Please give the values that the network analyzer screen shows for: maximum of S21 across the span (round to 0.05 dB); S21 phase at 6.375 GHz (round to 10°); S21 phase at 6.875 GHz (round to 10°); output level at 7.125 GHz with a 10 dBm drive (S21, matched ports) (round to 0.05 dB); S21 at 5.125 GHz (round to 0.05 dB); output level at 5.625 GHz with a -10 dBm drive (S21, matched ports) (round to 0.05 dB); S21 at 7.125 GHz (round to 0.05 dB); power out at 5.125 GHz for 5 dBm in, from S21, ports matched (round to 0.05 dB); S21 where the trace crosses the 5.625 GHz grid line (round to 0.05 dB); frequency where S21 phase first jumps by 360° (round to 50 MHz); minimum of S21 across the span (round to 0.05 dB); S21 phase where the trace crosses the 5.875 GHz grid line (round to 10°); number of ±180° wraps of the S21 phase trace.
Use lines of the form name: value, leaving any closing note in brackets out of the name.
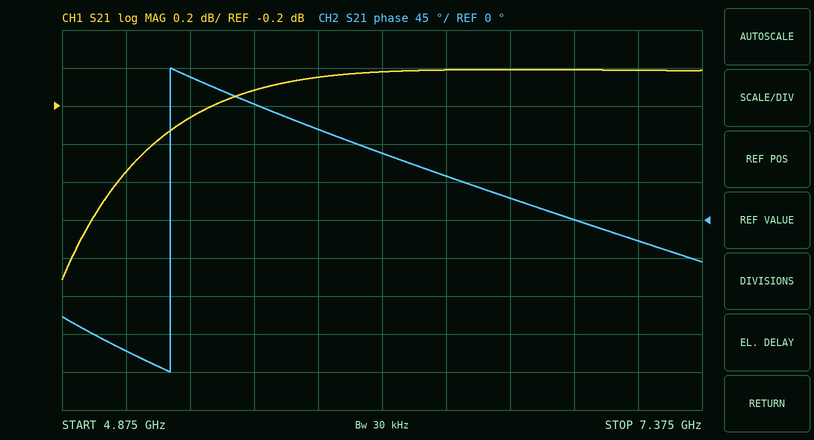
maximum of S21 across the span: 0.00 dB
S21 phase at 6.375 GHz: 50°
S21 phase at 6.875 GHz: 0°
output level at 7.125 GHz with a 10 dBm drive (S21, matched ports): 10.00 dBm
S21 at 5.125 GHz: -0.55 dB
output level at 5.625 GHz with a -10 dBm drive (S21, matched ports): -10.10 dBm
S21 at 7.125 GHz: 0.00 dB
power out at 5.125 GHz for 5 dBm in, from S21, ports matched: 4.45 dBm
S21 where the trace crosses the 5.625 GHz grid line: -0.10 dB
frequency where S21 phase first jumps by 360°: 5.30 GHz
minimum of S21 across the span: -1.10 dB
S21 phase where the trace crosses the 5.875 GHz grid line: 110°
number of ±180° wraps of the S21 phase trace: 1
